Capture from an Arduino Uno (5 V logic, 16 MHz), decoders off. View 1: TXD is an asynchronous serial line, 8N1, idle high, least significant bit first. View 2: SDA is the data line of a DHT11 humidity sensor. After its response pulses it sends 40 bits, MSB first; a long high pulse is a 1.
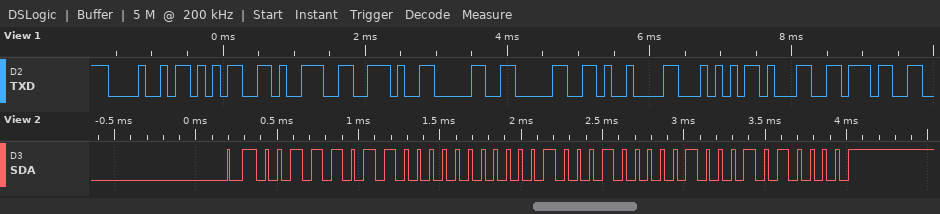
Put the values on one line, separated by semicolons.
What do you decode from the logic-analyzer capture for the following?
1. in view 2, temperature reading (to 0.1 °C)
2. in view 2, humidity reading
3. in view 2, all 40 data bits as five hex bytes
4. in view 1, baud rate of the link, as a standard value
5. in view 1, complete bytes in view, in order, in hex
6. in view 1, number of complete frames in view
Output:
17.4 °C; 59 %; 3B 00 11 04 50; 9600 baud; 48 35 39 2E 30 30 09 54 31 37; 10
